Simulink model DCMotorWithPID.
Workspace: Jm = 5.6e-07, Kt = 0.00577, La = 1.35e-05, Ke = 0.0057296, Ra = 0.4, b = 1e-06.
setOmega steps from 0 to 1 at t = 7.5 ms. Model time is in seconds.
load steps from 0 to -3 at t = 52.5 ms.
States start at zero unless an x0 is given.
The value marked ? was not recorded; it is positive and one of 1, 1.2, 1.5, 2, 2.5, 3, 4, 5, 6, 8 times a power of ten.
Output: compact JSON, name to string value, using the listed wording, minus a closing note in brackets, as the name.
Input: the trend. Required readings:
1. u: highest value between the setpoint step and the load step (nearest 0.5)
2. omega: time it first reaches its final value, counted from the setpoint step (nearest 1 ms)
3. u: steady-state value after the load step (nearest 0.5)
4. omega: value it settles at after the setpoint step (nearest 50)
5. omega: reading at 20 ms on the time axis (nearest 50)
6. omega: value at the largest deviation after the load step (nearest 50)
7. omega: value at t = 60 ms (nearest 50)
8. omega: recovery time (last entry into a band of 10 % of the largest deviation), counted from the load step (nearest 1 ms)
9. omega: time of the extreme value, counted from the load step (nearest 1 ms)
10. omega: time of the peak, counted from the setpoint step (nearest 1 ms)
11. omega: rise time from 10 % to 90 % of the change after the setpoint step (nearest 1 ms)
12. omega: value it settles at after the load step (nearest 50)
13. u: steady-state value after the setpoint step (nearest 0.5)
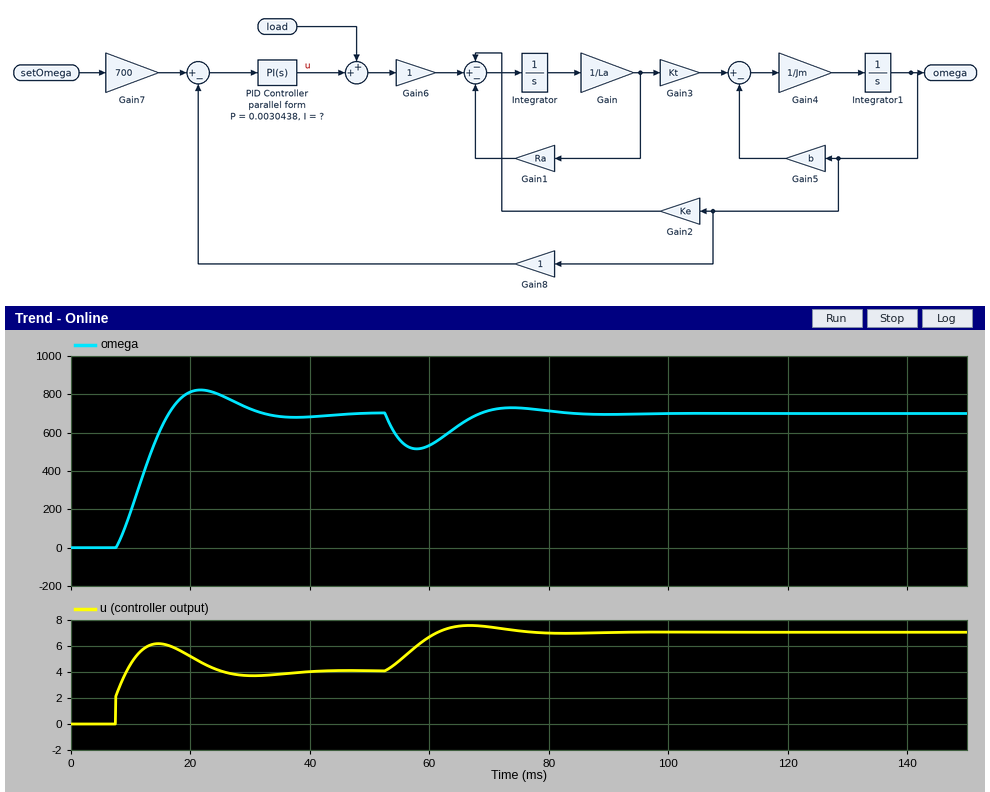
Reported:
{"u: highest value between the setpoint step and the load step": "6.0", "omega: time it first reaches its final value, counted from the setpoint step": "9 ms", "u: steady-state value after the load step": "7.0", "omega: value it settles at after the setpoint step": "700", "omega: reading at 20 ms on the time axis": "800", "omega: value at the largest deviation after the load step": "500", "omega: value at t = 60 ms": "550", "omega: recovery time (last entry into a band of 10 % of the largest deviation), counted from the load step": "26 ms", "omega: time of the extreme value, counted from the load step": "5 ms", "omega: time of the peak, counted from the setpoint step": "14 ms", "omega: rise time from 10 % to 90 % of the change after the setpoint step": "7 ms", "omega: value it settles at after the load step": "700", "u: steady-state value after the setpoint step": "4.0"}
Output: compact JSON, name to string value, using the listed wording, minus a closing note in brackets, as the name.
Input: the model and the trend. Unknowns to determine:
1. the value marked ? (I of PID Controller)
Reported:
{"the value marked ?": "2"}
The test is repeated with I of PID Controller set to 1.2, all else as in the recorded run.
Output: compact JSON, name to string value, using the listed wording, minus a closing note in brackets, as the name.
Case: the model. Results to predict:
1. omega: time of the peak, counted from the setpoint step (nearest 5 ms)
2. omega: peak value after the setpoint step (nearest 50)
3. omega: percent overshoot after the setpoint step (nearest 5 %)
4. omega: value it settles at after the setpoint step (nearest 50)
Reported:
{"omega: time of the peak, counted from the setpoint step": "20 ms", "omega: peak value after the setpoint step": "750", "omega: percent overshoot after the setpoint step": "10 %", "omega: value it settles at after the setpoint step": "700"}
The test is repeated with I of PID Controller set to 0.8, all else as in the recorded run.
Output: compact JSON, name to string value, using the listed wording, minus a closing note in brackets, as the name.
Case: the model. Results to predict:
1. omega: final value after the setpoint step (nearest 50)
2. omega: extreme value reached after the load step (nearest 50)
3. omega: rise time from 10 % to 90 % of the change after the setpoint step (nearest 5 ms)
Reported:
{"omega: final value after the setpoint step": "700", "omega: extreme value reached after the load step": "450", "omega: rise time from 10 % to 90 % of the change after the setpoint step": "15 ms"}
